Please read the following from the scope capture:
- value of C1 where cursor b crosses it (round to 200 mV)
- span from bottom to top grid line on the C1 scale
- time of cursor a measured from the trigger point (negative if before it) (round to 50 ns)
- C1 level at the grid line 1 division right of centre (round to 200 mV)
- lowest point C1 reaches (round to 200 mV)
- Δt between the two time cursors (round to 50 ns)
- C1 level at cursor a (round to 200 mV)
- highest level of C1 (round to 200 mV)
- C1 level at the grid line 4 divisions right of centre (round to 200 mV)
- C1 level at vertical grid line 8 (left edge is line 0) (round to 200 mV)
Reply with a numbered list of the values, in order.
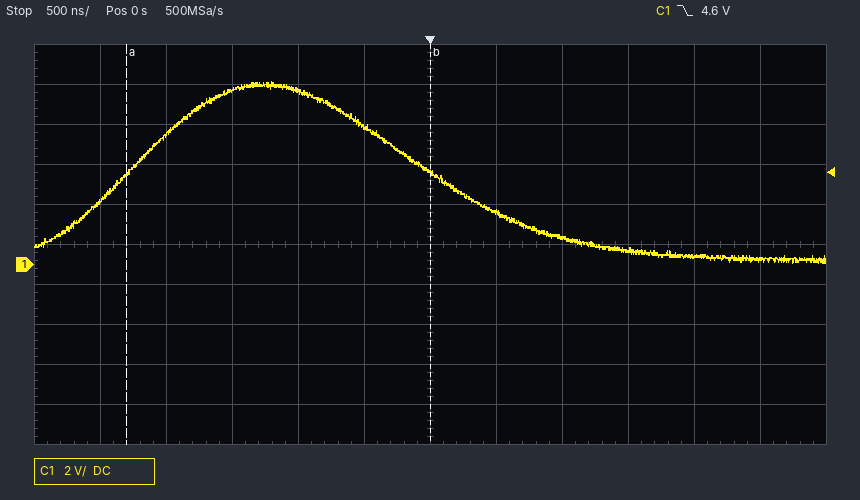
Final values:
1. 4.6 V
2. 20 V
3. -2.30 µs
4. 2.6 V
5. 0.0 V
6. 2.30 µs
7. 4.6 V
8. 9.2 V
9. 400 mV
10. 1.4 V
